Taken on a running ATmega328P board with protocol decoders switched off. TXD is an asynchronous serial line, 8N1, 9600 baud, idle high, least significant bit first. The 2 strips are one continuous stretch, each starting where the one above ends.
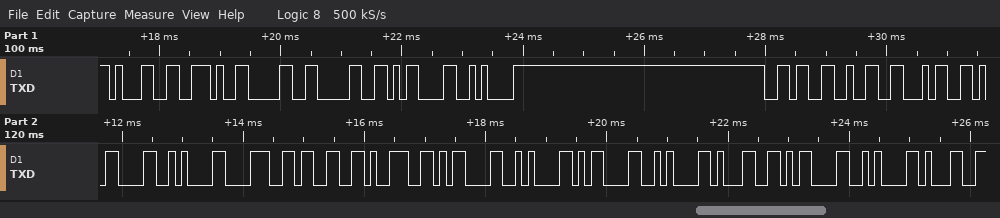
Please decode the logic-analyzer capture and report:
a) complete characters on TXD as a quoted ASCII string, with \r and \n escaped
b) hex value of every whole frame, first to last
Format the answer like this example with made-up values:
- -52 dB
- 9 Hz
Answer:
- "1.00\r\n624\r\n839\r\n\r\n1\r\n1"
- 31 2E 30 30 0D 0A 36 32 34 0D 0A 38 33 39 0D 0A 0D 0A 31 0D 0A 31
